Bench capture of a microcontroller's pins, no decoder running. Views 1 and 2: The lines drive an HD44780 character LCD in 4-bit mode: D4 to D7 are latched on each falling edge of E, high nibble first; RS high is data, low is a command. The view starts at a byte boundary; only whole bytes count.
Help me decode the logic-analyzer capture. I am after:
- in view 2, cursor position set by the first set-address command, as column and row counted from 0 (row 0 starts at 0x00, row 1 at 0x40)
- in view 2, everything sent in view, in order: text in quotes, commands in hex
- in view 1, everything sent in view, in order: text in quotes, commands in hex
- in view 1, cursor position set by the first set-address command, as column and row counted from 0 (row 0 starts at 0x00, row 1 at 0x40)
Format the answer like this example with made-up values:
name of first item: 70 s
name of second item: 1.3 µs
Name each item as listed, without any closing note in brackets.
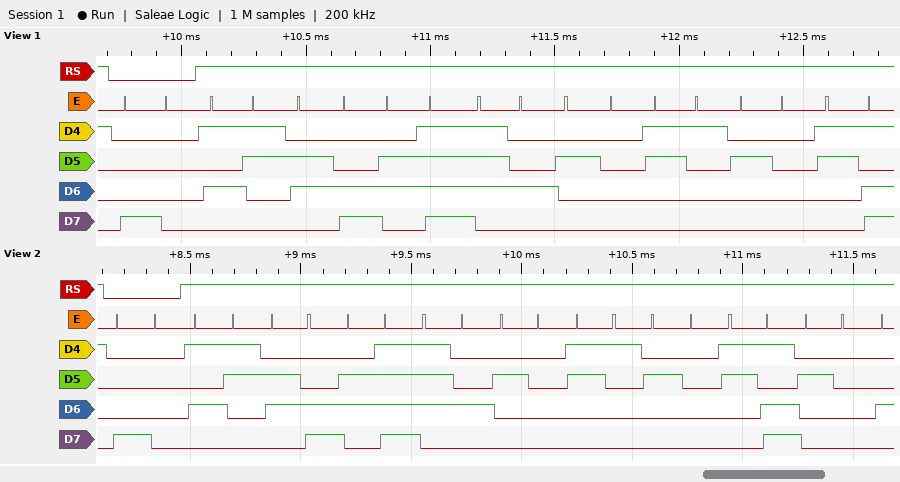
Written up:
in view 2, cursor position set by the first set-address command, as column and row counted from 0: column 0, row 0
in view 2, everything sent in view, in order: text in quotes, commands in hex: 0x80 "Slot 1 = "
in view 1, everything sent in view, in order: text in quotes, commands in hex: 0x80 "Slot 1 ="
in view 1, cursor position set by the first set-address command, as column and row counted from 0: column 0, row 0
